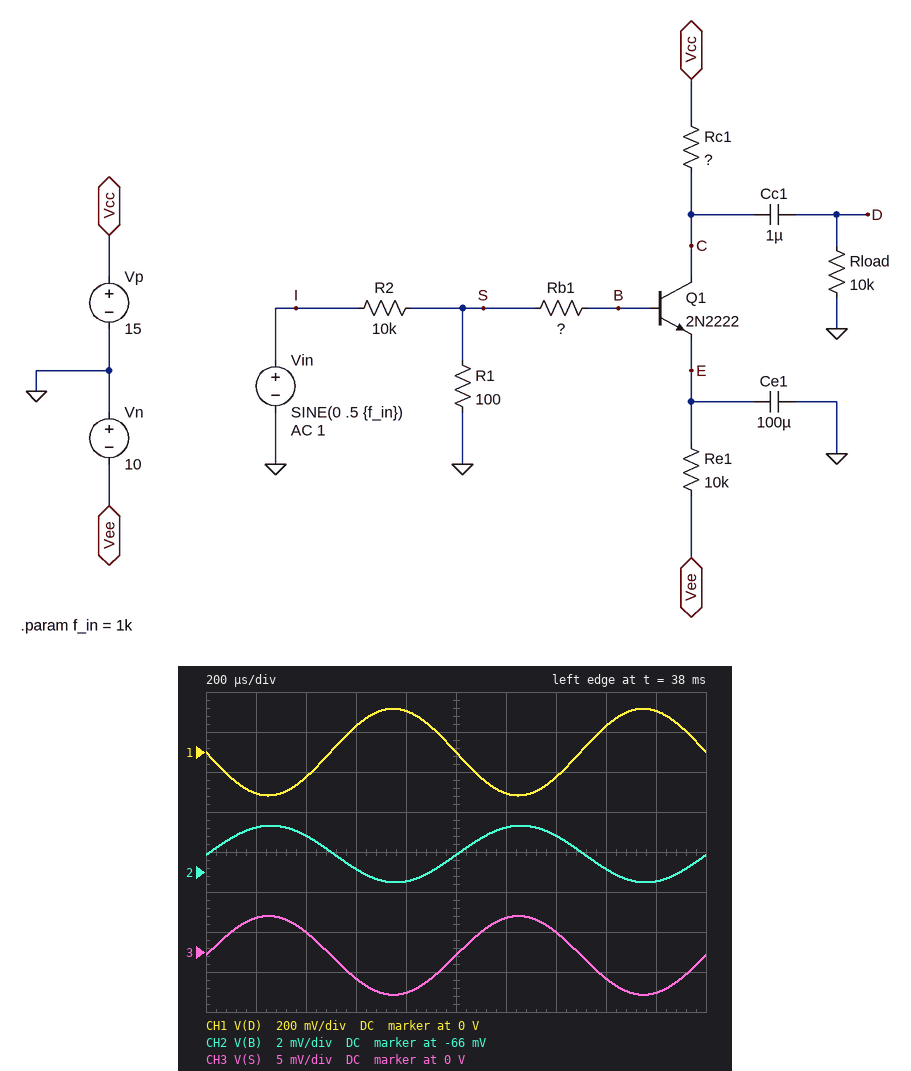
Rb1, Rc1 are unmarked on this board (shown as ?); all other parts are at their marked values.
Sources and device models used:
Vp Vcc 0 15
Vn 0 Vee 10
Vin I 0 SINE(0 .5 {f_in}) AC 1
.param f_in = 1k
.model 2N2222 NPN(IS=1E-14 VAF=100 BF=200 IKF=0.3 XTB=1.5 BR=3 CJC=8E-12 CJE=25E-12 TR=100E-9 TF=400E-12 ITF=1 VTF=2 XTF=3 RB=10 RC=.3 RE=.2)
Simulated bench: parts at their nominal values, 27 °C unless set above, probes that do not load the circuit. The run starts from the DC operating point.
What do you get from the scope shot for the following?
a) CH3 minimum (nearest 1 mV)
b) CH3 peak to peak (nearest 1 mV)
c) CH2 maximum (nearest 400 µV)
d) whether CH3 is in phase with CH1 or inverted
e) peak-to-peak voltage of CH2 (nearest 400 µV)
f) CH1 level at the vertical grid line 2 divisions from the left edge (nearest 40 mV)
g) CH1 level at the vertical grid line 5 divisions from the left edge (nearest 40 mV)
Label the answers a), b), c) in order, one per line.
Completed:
a) -5 mV
b) 10 mV
c) -63.6 mV
d) inverted
e) 2.8 mV
f) -120 mV
g) 0 V
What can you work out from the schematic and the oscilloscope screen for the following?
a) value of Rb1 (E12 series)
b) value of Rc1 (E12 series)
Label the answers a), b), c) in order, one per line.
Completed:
a) 15 kΩ
b) 8.2 kΩ
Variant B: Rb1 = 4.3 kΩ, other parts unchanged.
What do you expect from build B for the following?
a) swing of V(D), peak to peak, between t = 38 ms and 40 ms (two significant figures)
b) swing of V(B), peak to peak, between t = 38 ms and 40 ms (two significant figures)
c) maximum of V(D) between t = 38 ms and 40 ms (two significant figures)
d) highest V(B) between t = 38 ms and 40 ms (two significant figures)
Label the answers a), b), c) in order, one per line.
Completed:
a) 880 mV
b) 5.7 mV
c) 430 mV
d) -16 mV
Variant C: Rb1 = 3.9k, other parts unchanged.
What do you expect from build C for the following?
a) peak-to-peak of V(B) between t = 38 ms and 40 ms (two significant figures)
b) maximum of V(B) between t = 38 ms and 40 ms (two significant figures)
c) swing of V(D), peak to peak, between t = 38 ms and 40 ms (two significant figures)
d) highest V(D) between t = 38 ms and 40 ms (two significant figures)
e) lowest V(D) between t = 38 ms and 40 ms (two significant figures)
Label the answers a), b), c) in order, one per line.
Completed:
a) 6.0 mV
b) -14 mV
c) 910 mV
d) 450 mV
e) -460 mV
